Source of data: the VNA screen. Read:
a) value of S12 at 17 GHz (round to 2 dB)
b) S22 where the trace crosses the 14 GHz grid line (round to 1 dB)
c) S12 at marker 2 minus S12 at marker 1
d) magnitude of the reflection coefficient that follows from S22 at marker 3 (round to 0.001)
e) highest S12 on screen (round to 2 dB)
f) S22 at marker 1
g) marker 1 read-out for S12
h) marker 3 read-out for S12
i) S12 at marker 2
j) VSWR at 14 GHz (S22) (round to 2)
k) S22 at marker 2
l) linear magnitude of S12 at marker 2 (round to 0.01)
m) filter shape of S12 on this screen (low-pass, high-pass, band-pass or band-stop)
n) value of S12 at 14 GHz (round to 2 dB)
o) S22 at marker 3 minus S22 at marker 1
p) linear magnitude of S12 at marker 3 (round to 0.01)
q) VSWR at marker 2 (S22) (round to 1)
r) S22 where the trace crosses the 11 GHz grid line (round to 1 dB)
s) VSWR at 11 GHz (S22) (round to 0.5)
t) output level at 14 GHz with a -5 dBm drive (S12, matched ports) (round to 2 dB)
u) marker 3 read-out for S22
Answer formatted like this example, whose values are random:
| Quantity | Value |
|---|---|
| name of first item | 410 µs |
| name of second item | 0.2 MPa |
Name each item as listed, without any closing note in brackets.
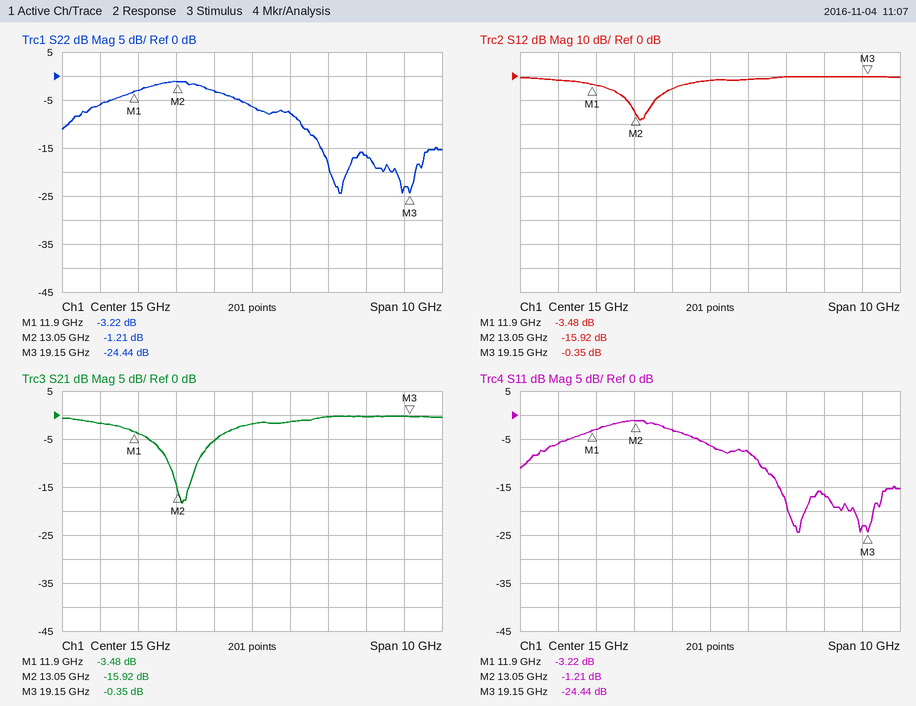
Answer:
| Quantity | Value |
|---|---|
| value of S12 at 17 GHz | 0 dB |
| S22 where the trace crosses the 14 GHz grid line | -3 dB |
| S12 at marker 2 minus S12 at marker 1 | -12.44 dB |
| magnitude of the reflection coefficient that follows from S22 at marker 3 | 0.060 |
| highest S12 on screen | 0 dB |
| S22 at marker 1 | -3.22 dB |
| marker 1 read-out for S12 | -3.48 dB |
| marker 3 read-out for S12 | -0.35 dB |
| S12 at marker 2 | -15.92 dB |
| VSWR at 14 GHz (S22) | 6 |
| S22 at marker 2 | -1.21 dB |
| linear magnitude of S12 at marker 2 | 0.16 |
| filter shape of S12 on this screen | band-stop |
| value of S12 at 14 GHz | -6 dB |
| S22 at marker 3 minus S22 at marker 1 | -21.22 dB |
| linear magnitude of S12 at marker 3 | 0.96 |
| VSWR at marker 2 (S22) | 14 |
| S22 where the trace crosses the 11 GHz grid line | -6 dB |
| VSWR at 11 GHz (S22) | 3.0 |
| output level at 14 GHz with a -5 dBm drive (S12, matched ports) | -10 dBm |
| marker 3 read-out for S22 | -24.44 dB |
